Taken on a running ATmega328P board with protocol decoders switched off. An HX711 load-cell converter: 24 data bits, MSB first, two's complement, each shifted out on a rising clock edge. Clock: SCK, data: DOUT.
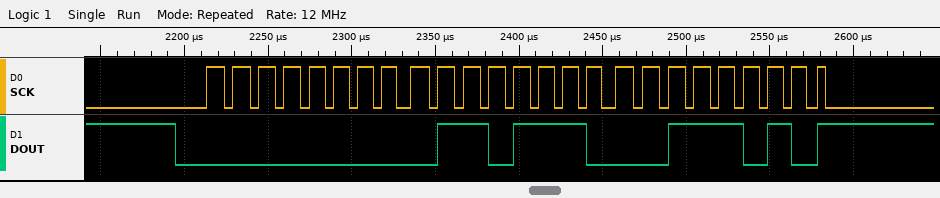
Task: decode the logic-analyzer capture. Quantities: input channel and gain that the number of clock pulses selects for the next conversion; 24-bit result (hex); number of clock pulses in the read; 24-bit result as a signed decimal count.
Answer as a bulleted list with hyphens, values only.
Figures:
- channel A, gain 128
- 0x006E3A
- 25
- 28218
